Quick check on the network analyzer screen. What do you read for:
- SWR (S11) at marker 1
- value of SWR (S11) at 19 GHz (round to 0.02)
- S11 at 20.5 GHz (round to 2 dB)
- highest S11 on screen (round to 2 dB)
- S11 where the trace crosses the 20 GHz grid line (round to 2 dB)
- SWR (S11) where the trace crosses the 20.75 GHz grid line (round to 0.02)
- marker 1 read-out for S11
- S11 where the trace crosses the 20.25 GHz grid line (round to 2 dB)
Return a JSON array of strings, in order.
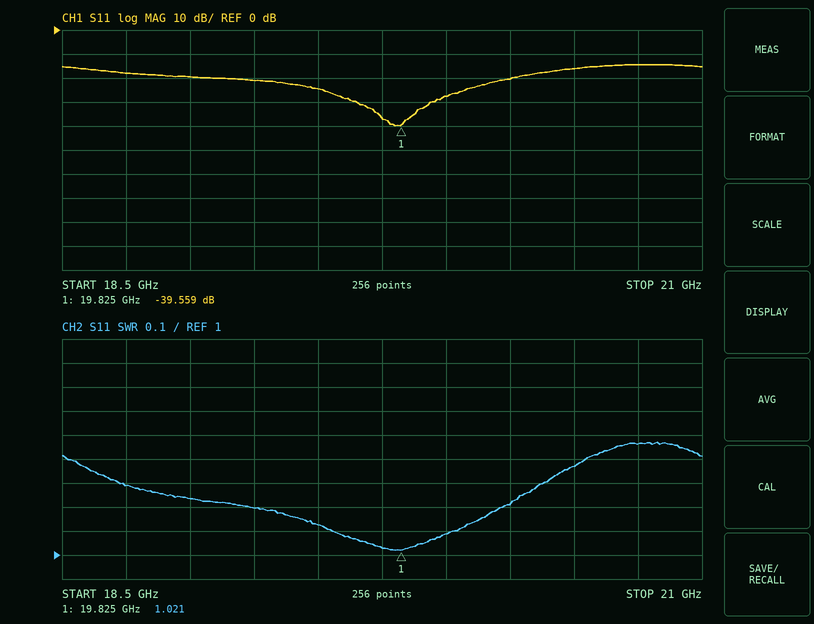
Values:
["1.021", "1.24", "-16 dB", "-14 dB", "-28 dB", "1.46", "-39.559 dB", "-20 dB"]
